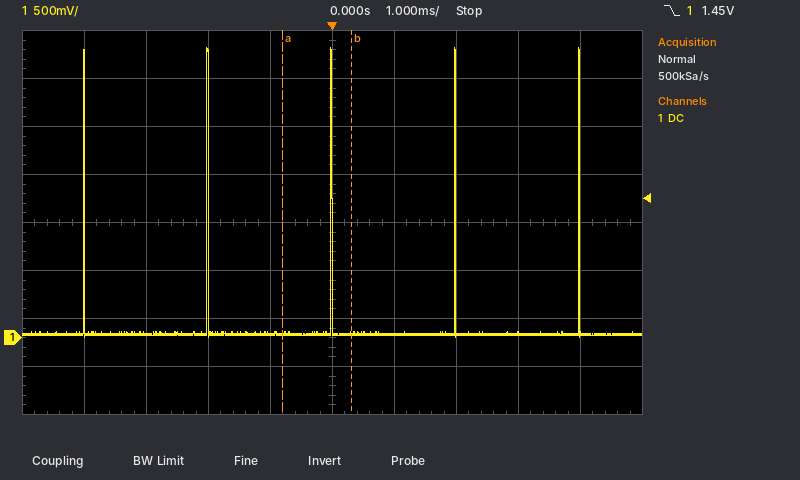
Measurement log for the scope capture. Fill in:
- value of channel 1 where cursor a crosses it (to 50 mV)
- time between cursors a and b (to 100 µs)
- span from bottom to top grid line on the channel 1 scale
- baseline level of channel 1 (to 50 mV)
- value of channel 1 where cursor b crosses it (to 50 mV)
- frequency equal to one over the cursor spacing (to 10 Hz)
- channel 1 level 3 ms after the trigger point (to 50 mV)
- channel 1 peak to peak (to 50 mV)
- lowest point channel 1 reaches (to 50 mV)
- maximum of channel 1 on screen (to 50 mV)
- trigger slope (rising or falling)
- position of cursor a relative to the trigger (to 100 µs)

50 mV
1.1 ms
4 V
50 mV
50 mV
910 Hz
50 mV
3.00 V
0 mV
3.00 V
falling
-800 µs
